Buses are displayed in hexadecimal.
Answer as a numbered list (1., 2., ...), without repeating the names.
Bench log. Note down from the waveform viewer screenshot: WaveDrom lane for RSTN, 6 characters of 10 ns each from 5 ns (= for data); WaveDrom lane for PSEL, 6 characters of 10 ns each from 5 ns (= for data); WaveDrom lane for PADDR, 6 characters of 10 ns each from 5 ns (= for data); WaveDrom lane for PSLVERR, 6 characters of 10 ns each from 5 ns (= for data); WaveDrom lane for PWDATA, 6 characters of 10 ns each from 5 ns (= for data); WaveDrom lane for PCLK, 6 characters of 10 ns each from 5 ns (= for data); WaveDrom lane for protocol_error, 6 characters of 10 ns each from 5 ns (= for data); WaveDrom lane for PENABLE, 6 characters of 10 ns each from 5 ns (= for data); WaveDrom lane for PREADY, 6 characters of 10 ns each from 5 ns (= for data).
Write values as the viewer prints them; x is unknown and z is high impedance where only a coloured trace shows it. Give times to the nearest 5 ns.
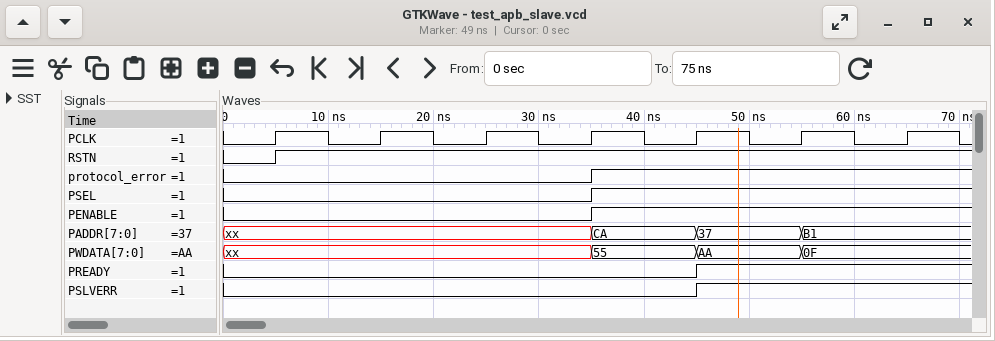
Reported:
1. {name: 'RSTN', wave: '1.....'}
2. {name: 'PSEL', wave: '0..1..'}
3. {name: 'PADDR', wave: 'x..===', data: 'CA 37 B1'}
4. {name: 'PSLVERR', wave: '0...1.'}
5. {name: 'PWDATA', wave: 'x..===', data: '55 AA 0F'}
6. {name: 'PCLK', wave: 'p.....'}
7. {name: 'protocol_error', wave: '0..1..'}
8. {name: 'PENABLE', wave: '0..1..'}
9. {name: 'PREADY', wave: '0...1.'}
